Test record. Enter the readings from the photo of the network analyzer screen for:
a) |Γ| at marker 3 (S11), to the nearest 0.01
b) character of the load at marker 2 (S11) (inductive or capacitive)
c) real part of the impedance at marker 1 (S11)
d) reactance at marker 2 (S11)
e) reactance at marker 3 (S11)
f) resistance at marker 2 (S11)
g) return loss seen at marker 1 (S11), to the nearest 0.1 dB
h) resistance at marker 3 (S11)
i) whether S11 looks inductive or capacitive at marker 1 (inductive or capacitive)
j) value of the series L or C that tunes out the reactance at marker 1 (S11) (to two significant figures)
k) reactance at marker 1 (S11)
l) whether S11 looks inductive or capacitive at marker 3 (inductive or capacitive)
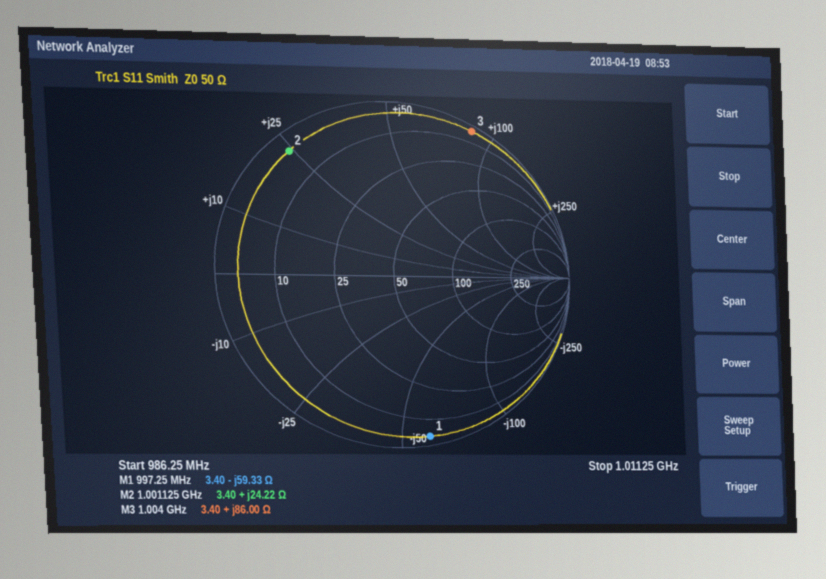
0.97
inductive
3.40 Ω
+24.22 Ω
+86.00 Ω
3.40 Ω
0.5 dB
3.40 Ω
capacitive
9.5 nH
-59.33 Ω
inductive
